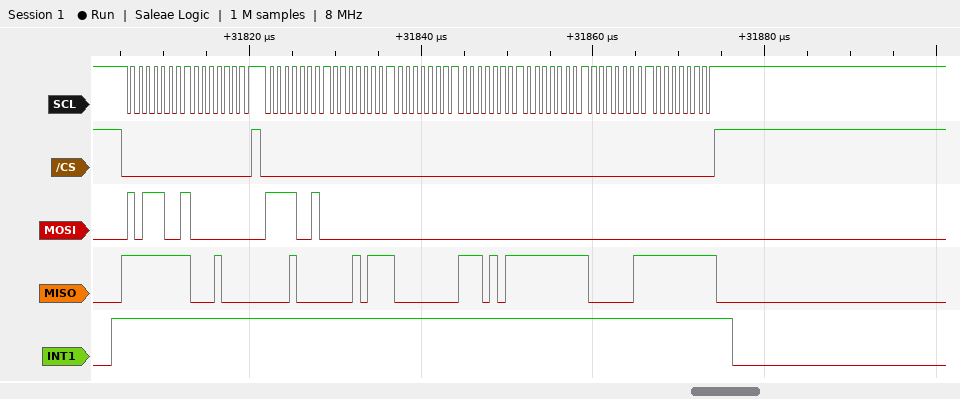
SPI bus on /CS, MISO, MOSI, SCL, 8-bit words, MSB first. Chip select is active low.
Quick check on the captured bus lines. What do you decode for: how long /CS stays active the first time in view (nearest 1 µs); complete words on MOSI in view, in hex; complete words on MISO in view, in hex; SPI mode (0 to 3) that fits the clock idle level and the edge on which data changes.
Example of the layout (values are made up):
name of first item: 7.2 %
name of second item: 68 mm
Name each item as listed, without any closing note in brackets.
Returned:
how long /CS stays active the first time in view: 15 µs
complete words on MOSI in view, in hex: B9, 00, F2, 00, 00, 00, 00, 00, 00
complete words on MISO in view, in hex: FF, 10, 10, 17, 00, EB, FF, 03, FF
SPI mode (0 to 3) that fits the clock idle level and the edge on which data changes: 3
